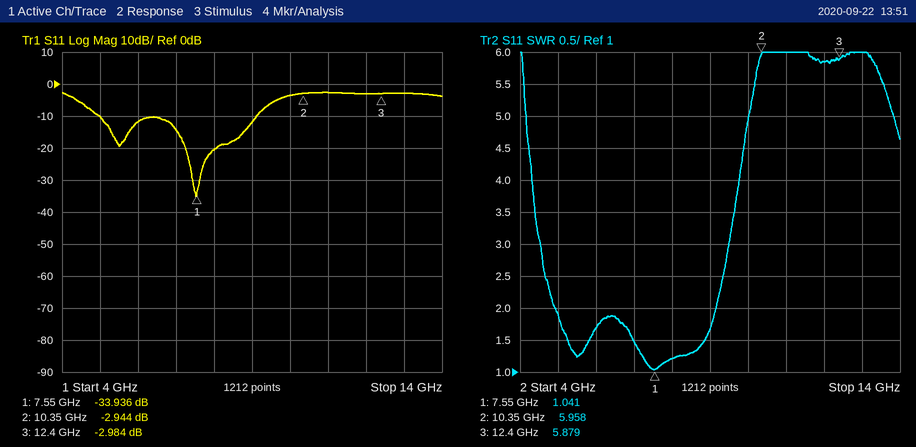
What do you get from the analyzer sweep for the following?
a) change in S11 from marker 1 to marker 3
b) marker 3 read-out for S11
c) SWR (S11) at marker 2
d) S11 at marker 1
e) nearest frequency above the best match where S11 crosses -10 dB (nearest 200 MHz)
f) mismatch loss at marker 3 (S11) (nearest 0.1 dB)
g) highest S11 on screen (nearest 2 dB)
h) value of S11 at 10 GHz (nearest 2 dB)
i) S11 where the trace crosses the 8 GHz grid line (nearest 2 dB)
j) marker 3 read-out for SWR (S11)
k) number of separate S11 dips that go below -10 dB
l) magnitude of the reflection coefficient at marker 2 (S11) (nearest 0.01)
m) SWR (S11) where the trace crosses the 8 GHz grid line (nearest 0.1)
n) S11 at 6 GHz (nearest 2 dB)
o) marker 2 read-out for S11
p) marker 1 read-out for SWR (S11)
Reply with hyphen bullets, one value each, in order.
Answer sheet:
- 30.952 dB
- -2.984 dB
- 5.958
- -33.936 dB
- 9.2 GHz
- 3.0 dB
- -2 dB
- -4 dB
- -20 dB
- 5.879
- 2
- 0.71
- 1.2
- -12 dB
- -2.944 dB
- 1.041
